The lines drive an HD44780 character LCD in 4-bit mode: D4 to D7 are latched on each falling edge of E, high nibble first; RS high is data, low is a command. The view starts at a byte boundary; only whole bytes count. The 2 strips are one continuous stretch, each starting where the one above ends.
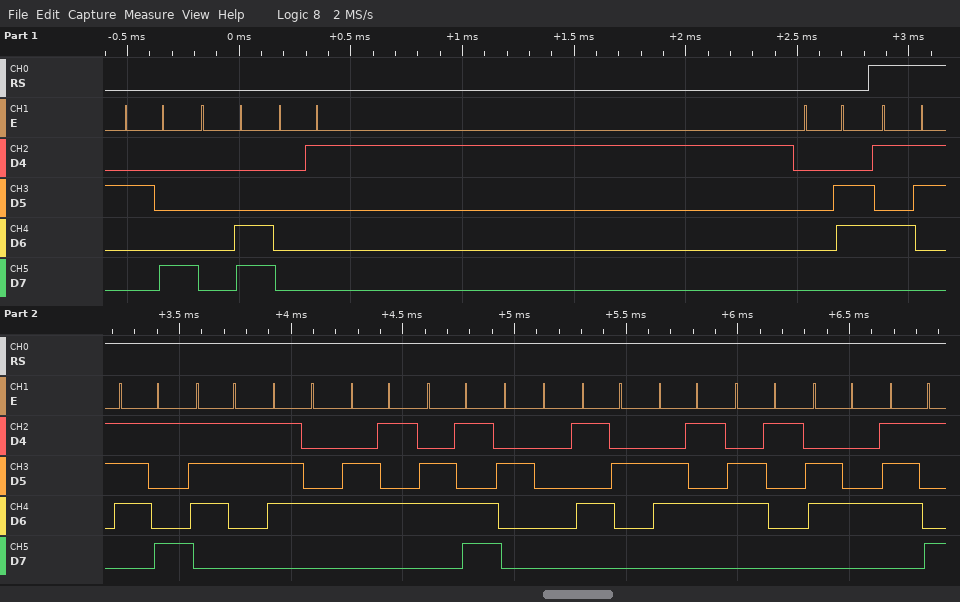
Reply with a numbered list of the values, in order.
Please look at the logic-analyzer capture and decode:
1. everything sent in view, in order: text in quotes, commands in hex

1. 0x28 0x0C 0x01 0x06 "System Ready"
